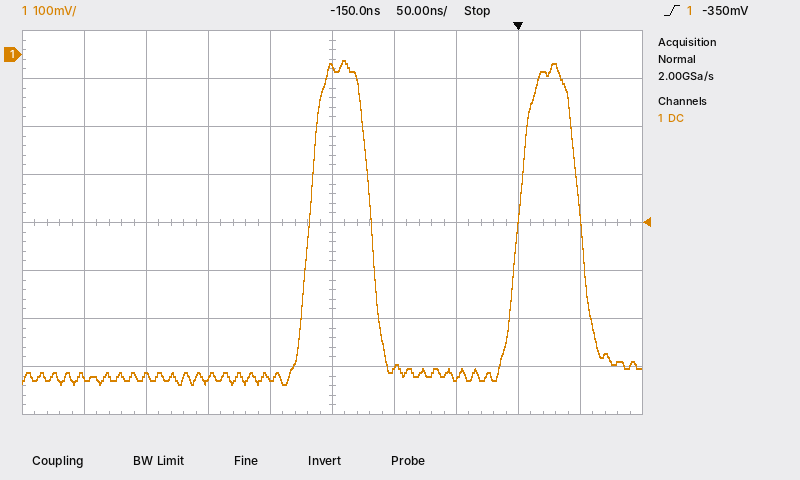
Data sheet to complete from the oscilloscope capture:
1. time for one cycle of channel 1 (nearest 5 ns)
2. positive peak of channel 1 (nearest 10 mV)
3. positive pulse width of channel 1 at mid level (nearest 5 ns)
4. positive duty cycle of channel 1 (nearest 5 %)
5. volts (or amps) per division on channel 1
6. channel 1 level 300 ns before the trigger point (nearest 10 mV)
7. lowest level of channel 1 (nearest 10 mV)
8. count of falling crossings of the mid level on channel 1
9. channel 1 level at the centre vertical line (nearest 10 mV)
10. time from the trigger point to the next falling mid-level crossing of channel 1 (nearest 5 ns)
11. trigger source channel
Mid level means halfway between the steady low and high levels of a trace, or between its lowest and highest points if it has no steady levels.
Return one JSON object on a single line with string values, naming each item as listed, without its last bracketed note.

{"time for one cycle of channel 1": "170 ns", "positive peak of channel 1": "-10 mV", "positive pulse width of channel 1 at mid level": "50 ns", "positive duty cycle of channel 1": "30 %", "volts (or amps) per division on channel 1": "100 mV", "channel 1 level 300 ns before the trigger point": "-670 mV", "lowest level of channel 1": "-690 mV", "count of falling crossings of the mid level on channel 1": "2", "channel 1 level at the centre vertical line": "-30 mV", "time from the trigger point to the next falling mid-level crossing of channel 1": "50 ns", "trigger source channel": "channel 1"}
